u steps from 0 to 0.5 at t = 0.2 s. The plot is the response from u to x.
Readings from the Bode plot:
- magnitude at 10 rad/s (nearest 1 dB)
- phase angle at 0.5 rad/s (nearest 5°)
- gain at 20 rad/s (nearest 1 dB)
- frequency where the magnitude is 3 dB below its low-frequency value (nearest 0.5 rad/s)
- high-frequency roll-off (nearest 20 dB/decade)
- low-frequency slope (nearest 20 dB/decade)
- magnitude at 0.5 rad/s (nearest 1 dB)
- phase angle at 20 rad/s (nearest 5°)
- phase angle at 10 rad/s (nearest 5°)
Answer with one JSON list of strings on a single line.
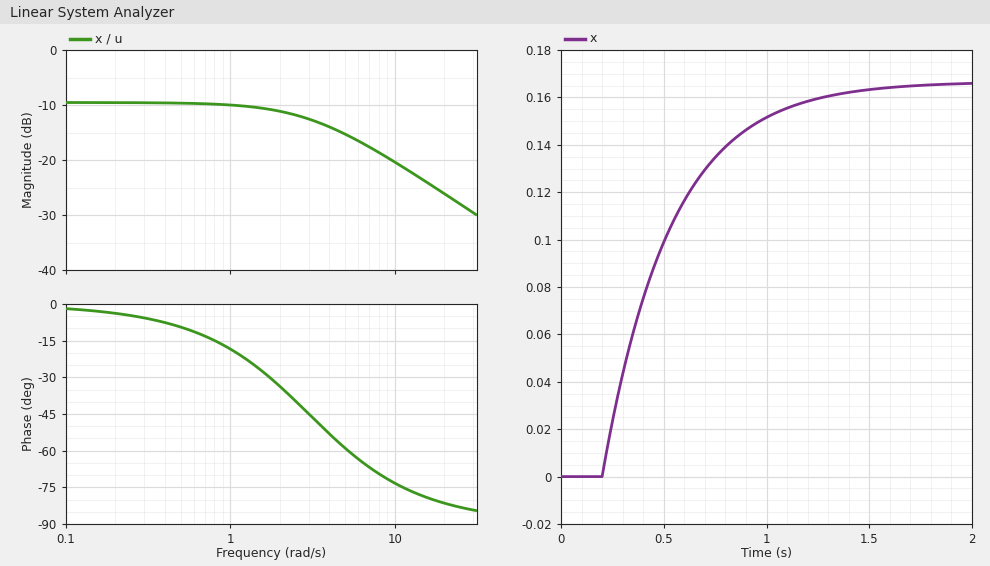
["-20 dB", "-10°", "-26 dB", "3.0 rad/s", "-20 dB/decade", "0 dB/decade", "-10 dB", "-80°", "-75°"]
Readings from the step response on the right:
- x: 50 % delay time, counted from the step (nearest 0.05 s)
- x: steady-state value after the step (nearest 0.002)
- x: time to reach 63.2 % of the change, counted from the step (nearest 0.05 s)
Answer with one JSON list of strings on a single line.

["0.25 s", "0.166", "0.35 s"]
